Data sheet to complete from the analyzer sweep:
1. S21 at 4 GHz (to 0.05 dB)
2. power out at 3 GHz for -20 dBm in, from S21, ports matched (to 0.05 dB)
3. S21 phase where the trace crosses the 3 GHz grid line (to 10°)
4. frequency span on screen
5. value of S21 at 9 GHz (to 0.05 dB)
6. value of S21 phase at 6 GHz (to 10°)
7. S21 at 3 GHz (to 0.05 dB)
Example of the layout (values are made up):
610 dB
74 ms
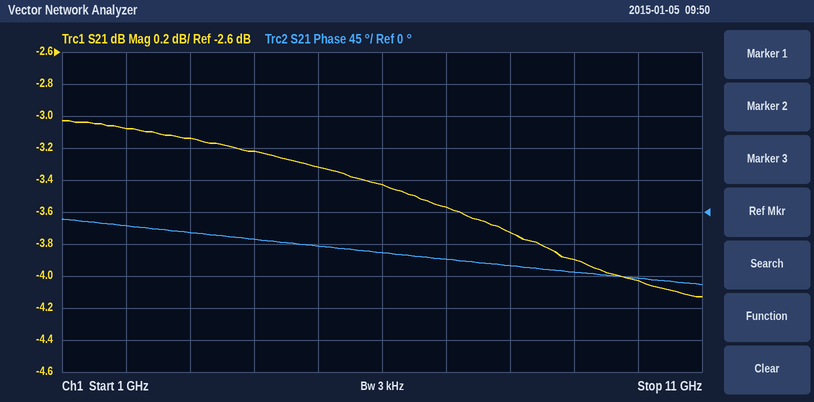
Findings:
-3.20 dB
-23.15 dBm
-30°
10 GHz
-3.90 dB
-60°
-3.15 dB
